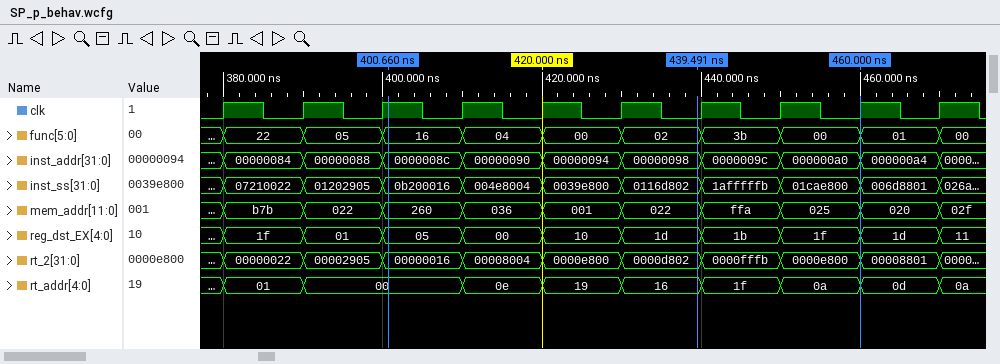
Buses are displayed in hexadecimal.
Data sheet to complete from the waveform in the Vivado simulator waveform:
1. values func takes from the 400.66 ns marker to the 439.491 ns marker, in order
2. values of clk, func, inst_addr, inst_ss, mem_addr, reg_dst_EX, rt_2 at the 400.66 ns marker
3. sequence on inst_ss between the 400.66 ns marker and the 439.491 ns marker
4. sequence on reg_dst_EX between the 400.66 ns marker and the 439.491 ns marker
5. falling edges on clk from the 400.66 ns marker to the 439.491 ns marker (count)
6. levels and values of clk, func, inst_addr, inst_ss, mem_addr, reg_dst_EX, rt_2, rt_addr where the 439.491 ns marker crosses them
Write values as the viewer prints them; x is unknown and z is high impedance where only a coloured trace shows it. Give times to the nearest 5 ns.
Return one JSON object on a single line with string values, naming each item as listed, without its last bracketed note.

{"values func takes from the 400.66 ns marker to the 439.491 ns marker, in order": "16, 04, 00, 02", "values of clk, func, inst_addr, inst_ss, mem_addr, reg_dst_EX, rt_2 at the 400.66 ns marker": "clk=1, func=16, inst_addr=0000008c, inst_ss=0b200016, mem_addr=260, reg_dst_EX=05, rt_2=00000016", "sequence on inst_ss between the 400.66 ns marker and the 439.491 ns marker": "0b200016, 004e8004, 0039e800, 0116d802", "sequence on reg_dst_EX between the 400.66 ns marker and the 439.491 ns marker": "05, 00, 10, 1d", "falling edges on clk from the 400.66 ns marker to the 439.491 ns marker": "4", "levels and values of clk, func, inst_addr, inst_ss, mem_addr, reg_dst_EX, rt_2, rt_addr where the 439.491 ns marker crosses them": "clk=0, func=02, inst_addr=00000098, inst_ss=0116d802, mem_addr=022, reg_dst_EX=1d, rt_2=0000d802, rt_addr=16"}
